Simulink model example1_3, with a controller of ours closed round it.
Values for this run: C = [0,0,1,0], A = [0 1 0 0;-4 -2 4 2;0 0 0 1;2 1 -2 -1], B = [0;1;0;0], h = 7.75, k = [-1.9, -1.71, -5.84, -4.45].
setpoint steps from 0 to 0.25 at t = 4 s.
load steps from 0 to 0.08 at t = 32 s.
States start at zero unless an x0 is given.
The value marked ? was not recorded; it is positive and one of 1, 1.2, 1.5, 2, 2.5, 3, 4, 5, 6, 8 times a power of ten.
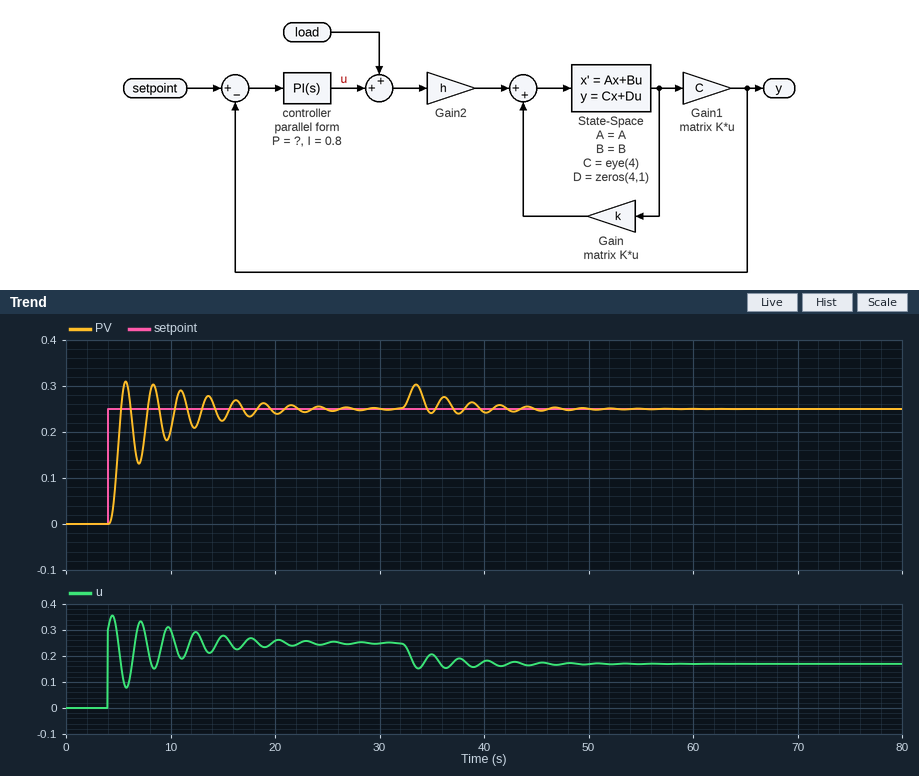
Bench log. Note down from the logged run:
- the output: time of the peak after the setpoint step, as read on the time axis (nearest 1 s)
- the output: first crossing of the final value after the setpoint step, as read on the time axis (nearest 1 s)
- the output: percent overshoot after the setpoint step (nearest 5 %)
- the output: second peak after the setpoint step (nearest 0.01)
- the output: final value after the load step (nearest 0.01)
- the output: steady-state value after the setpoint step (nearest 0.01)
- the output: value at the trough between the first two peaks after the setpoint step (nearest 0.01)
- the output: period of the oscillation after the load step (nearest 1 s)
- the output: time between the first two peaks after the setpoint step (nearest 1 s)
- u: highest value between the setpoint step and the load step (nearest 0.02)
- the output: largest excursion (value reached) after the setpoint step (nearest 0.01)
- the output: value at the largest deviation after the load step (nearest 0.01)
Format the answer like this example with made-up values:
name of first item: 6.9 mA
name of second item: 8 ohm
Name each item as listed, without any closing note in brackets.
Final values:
the output: time of the peak after the setpoint step, as read on the time axis: 6 s
the output: first crossing of the final value after the setpoint step, as read on the time axis: 5 s
the output: percent overshoot after the setpoint step: 25 %
the output: second peak after the setpoint step: 0.30
the output: final value after the load step: 0.25
the output: steady-state value after the setpoint step: 0.25
the output: value at the trough between the first two peaks after the setpoint step: 0.13
the output: period of the oscillation after the load step: 3 s
the output: time between the first two peaks after the setpoint step: 3 s
u: highest value between the setpoint step and the load step: 0.36
the output: largest excursion (value reached) after the setpoint step: 0.31
the output: value at the largest deviation after the load step: 0.30
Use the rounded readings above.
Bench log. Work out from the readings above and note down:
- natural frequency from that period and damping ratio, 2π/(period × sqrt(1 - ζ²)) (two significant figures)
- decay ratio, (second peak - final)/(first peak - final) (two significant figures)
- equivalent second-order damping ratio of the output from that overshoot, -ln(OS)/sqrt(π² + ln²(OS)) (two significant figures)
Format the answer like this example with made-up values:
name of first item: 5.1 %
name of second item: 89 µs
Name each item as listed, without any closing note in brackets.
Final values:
natural frequency from that period and damping ratio, 2π/(period × sqrt(1 - ζ²)): 2.3 rad/s
decay ratio, (second peak - final)/(first peak - final): 0.83
equivalent second-order damping ratio of the output from that overshoot, -ln(OS)/sqrt(π² + ln²(OS)): 0.40
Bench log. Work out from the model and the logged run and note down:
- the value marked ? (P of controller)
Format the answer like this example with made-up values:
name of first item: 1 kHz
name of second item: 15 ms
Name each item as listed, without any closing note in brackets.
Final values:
the value marked ?: 1.2
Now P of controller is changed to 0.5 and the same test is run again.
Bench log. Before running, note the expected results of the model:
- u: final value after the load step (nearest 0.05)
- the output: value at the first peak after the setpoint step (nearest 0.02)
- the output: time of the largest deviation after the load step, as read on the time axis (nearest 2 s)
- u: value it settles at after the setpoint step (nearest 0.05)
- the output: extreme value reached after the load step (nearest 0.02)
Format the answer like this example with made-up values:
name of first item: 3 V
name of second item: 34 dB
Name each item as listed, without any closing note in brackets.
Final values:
u: final value after the load step: 0.15
the output: value at the first peak after the setpoint step: 0.28
the output: time of the largest deviation after the load step, as read on the time axis: 34 s
u: value it settles at after the setpoint step: 0.25
the output: extreme value reached after the load step: 0.32
